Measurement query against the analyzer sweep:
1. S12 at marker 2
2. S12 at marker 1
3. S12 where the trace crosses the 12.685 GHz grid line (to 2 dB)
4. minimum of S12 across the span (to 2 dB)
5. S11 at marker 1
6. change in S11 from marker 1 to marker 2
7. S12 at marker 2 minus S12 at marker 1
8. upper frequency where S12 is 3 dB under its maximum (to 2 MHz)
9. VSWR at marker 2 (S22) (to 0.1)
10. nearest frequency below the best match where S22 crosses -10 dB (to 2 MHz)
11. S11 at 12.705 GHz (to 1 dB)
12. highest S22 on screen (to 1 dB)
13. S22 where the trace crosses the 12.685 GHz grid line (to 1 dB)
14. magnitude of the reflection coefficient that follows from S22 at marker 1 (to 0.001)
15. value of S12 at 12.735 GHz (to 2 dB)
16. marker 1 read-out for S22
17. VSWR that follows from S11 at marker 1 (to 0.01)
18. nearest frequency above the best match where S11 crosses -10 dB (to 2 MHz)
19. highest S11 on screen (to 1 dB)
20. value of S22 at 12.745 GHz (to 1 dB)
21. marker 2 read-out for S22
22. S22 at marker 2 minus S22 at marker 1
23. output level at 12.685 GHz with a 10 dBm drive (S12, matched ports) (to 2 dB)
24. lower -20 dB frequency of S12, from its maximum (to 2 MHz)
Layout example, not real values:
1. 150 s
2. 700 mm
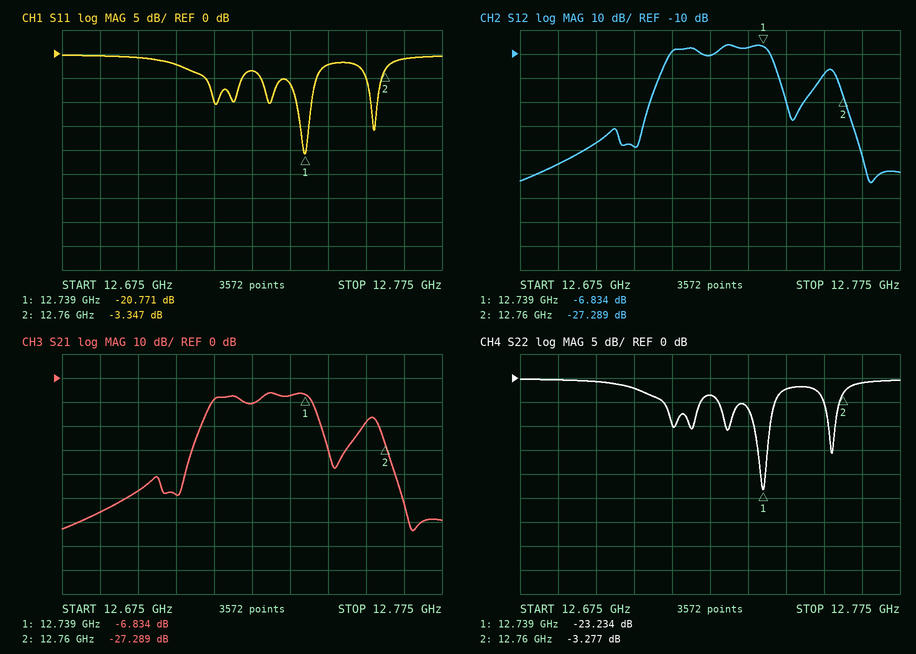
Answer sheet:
1. -27.289 dB
2. -6.834 dB
3. -56 dB
4. -64 dB
5. -20.771 dB
6. 17.424 dB
7. -20.455 dB
8. 12.740 GHz
9. 5.4
10. 12.736 GHz
11. -2 dB
12. 0 dB
13. 0 dB
14. 0.069
15. -8 dB
16. -23.234 dB
17. 1.20
18. 12.740 GHz
19. 0 dB
20. -2 dB
21. -3.277 dB
22. 19.957 dB
23. -46 dBm
24. 12.710 GHz
